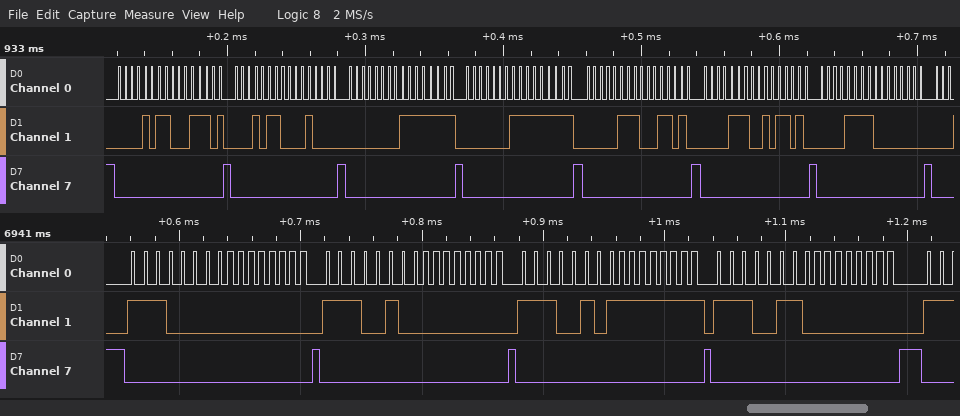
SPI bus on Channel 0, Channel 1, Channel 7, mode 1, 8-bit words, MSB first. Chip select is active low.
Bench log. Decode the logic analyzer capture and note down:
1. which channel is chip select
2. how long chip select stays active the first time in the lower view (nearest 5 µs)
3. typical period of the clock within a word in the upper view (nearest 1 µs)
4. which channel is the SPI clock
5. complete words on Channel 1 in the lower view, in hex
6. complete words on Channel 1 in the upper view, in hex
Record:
Channel 7
155 µs
5 µs
Channel 0
E0, 00, E4, 00, E5, FF, E6, 00
0B, 1D, 16, 10, 00, FF, 01, FF, 07, 1A, 0E, 5A, 0F, 00
